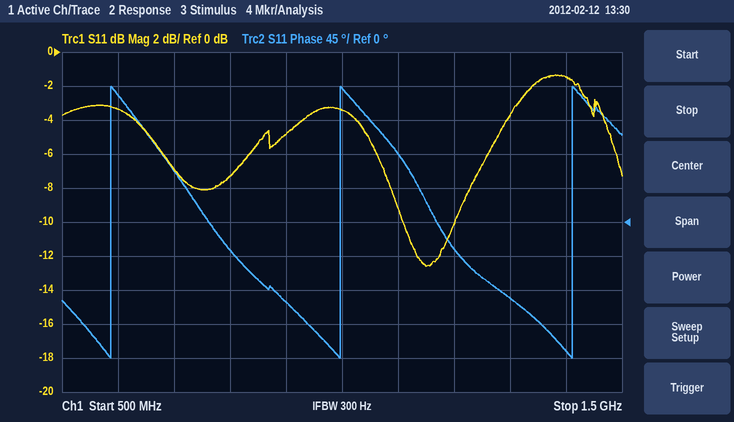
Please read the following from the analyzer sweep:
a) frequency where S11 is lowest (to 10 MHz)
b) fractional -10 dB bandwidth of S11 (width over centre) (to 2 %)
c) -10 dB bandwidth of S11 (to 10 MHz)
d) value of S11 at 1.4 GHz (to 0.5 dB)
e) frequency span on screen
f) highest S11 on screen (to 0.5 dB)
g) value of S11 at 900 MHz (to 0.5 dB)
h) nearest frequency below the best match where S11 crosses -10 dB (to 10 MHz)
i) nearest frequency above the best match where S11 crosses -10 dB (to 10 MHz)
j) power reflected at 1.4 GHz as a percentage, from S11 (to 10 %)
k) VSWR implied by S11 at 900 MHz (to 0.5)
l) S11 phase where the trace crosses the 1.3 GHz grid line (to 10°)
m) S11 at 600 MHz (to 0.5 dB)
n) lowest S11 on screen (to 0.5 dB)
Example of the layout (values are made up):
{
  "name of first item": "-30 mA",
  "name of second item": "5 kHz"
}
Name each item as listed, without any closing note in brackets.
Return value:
{
  "frequency where S11 is lowest": "1.15 GHz",
  "fractional -10 dB bandwidth of S11 (width over centre)": "8 %",
  "-10 dB bandwidth of S11": "90 MHz",
  "value of S11 at 1.4 GHz": "-1.5 dB",
  "frequency span on screen": "1 GHz",
  "highest S11 on screen": "-1.5 dB",
  "value of S11 at 900 MHz": "-5.0 dB",
  "nearest frequency below the best match where S11 crosses -10 dB": "1.11 GHz",
  "nearest frequency above the best match where S11 crosses -10 dB": "1.20 GHz",
  "power reflected at 1.4 GHz as a percentage, from S11": "70 %",
  "VSWR implied by S11 at 900 MHz": "3.5",
  "S11 phase where the trace crosses the 1.3 GHz grid line": "-100°",
  "S11 at 600 MHz": "-3.5 dB",
  "lowest S11 on screen": "-12.5 dB"
}
